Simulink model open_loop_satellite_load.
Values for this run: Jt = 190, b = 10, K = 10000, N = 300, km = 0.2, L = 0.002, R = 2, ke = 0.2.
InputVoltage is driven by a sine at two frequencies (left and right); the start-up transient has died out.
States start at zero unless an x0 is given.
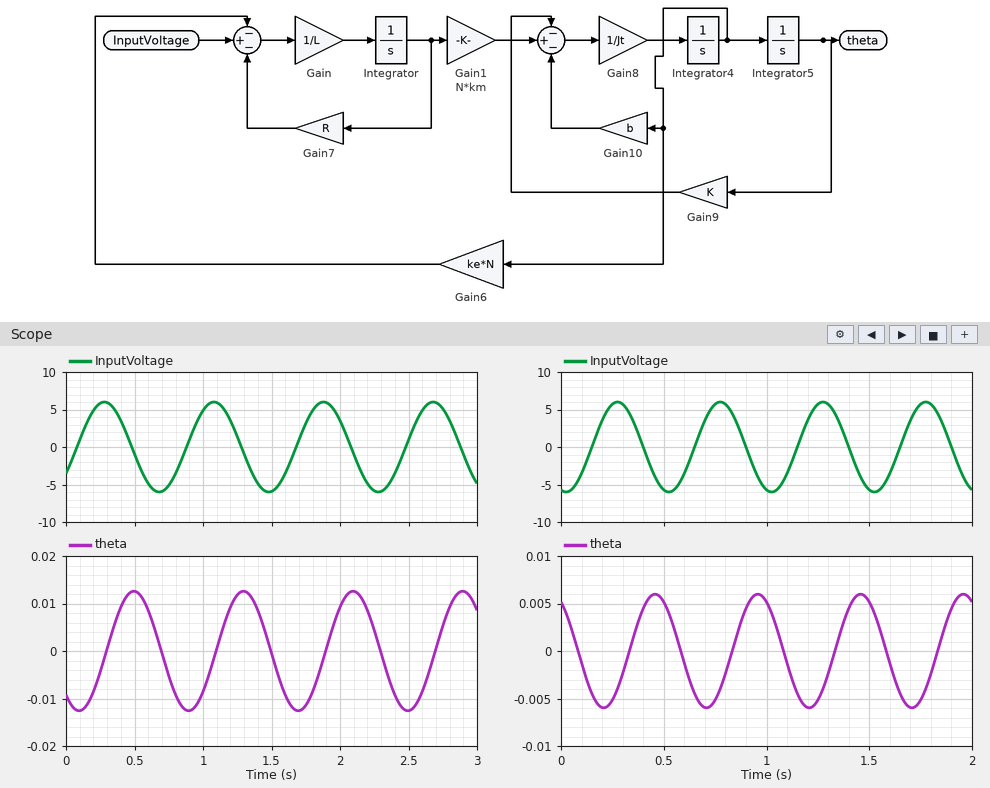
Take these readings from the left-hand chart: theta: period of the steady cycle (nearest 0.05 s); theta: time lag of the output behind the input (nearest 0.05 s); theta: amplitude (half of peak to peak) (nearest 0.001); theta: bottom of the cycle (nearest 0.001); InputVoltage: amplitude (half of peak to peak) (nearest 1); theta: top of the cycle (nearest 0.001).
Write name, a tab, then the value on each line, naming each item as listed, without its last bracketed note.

theta: period of the steady cycle	0.80 s
theta: time lag of the output behind the input	0.20 s
theta: amplitude (half of peak to peak)	0.013
theta: bottom of the cycle	-0.013
InputVoltage: amplitude (half of peak to peak)	6
theta: top of the cycle	0.013
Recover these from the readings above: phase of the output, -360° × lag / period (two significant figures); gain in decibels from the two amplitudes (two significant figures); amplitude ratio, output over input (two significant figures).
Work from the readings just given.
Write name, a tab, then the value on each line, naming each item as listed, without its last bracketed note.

phase of the output, -360° × lag / period	-90°
gain in decibels from the two amplitudes	-53 dB
amplitude ratio, output over input	0.0022
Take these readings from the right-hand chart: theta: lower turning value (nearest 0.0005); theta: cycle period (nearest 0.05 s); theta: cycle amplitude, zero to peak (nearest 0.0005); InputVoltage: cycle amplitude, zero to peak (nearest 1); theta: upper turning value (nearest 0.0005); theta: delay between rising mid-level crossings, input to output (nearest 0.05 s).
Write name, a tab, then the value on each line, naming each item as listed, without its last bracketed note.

theta: lower turning value	-0.0060
theta: cycle period	0.50 s
theta: cycle amplitude, zero to peak	0.0060
InputVoltage: cycle amplitude, zero to peak	6
theta: upper turning value	0.0060
theta: delay between rising mid-level crossings, input to output	0.20 s
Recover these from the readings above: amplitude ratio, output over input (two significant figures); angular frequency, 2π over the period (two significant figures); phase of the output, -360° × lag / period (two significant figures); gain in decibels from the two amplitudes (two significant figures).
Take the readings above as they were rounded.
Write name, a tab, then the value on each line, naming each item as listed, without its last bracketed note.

amplitude ratio, output over input	0.0010
angular frequency, 2π over the period	13 rad/s
phase of the output, -360° × lag / period	-140°
gain in decibels from the two amplitudes	-60 dB
